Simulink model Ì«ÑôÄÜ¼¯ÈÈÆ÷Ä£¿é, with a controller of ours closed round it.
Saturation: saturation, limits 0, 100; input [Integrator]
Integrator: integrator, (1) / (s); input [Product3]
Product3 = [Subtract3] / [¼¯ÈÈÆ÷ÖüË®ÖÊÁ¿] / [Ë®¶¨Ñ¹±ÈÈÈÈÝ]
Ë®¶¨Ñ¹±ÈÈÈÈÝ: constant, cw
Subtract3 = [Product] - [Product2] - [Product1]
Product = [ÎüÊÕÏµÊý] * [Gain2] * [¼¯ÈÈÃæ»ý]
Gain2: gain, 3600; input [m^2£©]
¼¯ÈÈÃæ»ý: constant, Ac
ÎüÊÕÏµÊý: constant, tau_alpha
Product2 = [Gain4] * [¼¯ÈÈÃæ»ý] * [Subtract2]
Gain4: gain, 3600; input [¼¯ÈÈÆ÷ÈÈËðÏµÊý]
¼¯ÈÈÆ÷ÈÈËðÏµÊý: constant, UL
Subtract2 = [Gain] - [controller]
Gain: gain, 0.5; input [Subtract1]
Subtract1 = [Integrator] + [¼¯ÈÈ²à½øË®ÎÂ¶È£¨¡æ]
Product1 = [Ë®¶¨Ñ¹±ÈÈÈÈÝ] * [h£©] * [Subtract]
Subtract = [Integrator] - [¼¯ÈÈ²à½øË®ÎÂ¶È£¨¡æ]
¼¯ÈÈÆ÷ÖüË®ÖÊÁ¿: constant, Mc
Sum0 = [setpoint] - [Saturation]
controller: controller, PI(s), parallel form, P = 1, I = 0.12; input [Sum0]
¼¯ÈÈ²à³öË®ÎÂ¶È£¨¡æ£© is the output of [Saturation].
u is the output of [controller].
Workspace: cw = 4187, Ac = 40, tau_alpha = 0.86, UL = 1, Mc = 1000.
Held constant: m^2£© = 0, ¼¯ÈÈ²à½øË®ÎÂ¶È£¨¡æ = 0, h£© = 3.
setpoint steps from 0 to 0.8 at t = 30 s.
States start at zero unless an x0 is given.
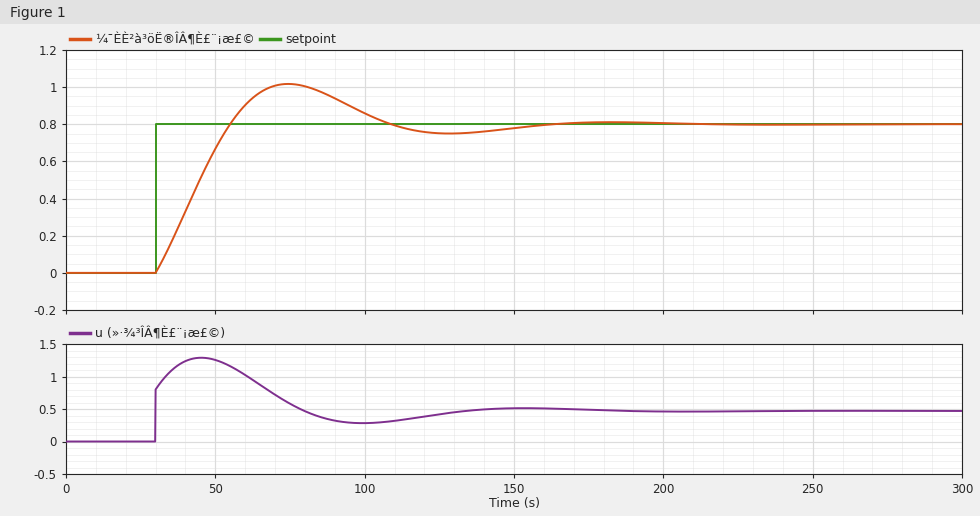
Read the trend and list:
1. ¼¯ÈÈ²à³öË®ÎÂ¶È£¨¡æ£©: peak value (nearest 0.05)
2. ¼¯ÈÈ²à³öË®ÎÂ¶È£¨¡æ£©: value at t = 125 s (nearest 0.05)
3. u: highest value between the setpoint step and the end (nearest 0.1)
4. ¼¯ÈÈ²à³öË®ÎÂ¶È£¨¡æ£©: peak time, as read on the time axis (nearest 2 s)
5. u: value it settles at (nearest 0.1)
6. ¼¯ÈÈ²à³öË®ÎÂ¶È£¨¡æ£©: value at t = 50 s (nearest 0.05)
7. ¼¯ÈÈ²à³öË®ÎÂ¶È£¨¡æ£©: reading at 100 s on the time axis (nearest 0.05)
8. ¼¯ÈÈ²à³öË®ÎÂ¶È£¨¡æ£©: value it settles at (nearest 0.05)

1.00
0.75
1.3
74 s
0.5
0.65
0.85
0.80
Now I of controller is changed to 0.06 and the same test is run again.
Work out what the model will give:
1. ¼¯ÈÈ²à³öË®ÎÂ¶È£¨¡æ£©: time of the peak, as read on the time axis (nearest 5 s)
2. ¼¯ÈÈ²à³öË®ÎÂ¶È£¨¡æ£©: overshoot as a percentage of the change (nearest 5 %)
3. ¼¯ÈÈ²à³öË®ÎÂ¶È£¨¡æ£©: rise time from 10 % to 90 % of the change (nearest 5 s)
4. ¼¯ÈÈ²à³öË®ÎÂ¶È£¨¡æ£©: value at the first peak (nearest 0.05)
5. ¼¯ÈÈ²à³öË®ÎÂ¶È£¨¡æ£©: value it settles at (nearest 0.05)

95 s
15 %
30 s
0.90
0.80
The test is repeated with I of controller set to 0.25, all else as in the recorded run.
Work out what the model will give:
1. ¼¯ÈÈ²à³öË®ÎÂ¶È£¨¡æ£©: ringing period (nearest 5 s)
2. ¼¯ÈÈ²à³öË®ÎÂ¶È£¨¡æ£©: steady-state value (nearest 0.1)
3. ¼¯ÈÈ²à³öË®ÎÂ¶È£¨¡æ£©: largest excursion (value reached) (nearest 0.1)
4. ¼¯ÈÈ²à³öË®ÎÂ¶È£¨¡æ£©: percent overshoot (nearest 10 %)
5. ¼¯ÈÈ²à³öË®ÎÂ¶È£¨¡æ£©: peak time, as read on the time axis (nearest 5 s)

70 s
0.8
1.1
40 %
60 s
